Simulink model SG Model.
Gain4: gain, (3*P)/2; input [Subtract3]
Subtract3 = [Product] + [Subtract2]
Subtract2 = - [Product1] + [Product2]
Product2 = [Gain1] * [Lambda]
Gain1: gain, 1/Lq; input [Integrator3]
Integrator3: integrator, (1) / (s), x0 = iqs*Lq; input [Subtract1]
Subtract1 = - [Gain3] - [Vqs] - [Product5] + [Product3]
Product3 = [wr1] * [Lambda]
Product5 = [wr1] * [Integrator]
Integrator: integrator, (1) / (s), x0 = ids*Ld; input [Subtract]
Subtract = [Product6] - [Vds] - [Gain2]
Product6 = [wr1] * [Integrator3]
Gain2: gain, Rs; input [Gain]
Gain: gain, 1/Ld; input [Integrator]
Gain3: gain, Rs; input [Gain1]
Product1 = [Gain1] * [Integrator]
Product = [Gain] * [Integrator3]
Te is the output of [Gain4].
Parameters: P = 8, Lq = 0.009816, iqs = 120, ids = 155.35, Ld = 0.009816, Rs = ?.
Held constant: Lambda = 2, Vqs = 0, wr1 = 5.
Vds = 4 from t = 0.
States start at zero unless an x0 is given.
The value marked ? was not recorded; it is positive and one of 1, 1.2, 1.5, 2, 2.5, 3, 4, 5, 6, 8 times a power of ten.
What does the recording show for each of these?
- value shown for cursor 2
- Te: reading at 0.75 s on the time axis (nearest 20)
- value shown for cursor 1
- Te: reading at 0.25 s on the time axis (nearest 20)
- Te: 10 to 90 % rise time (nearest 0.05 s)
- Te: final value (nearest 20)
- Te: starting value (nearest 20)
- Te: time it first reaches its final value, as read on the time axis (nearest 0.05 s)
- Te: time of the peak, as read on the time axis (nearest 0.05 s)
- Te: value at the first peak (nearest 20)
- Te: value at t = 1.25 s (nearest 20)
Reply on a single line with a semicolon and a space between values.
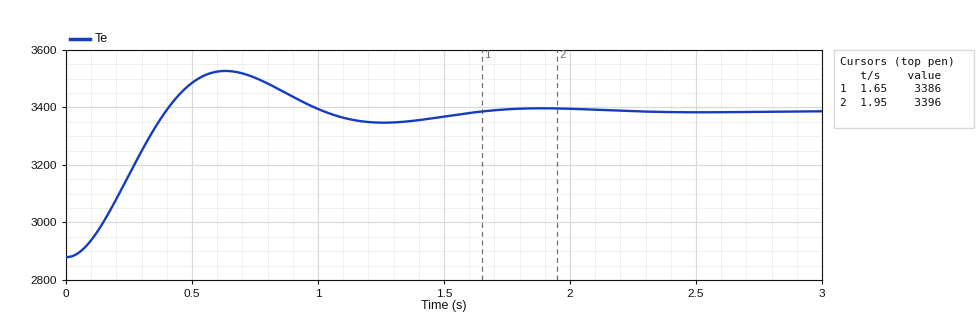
3396; 3500; 3386; 3160; 0.25 s; 3380; 2880; 0.40 s; 0.65 s; 3520; 3340
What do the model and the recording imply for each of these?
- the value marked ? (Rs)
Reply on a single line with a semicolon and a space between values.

0.02
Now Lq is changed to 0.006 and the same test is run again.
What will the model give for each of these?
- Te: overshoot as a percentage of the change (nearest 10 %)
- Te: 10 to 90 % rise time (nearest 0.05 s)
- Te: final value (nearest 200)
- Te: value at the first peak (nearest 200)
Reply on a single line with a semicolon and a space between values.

20 %; 0.25 s; 4000; 4400
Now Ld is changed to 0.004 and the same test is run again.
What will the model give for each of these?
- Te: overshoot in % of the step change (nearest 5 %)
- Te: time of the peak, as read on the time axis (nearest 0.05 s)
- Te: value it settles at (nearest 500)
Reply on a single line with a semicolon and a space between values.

15 %; 0.55 s; 9000
